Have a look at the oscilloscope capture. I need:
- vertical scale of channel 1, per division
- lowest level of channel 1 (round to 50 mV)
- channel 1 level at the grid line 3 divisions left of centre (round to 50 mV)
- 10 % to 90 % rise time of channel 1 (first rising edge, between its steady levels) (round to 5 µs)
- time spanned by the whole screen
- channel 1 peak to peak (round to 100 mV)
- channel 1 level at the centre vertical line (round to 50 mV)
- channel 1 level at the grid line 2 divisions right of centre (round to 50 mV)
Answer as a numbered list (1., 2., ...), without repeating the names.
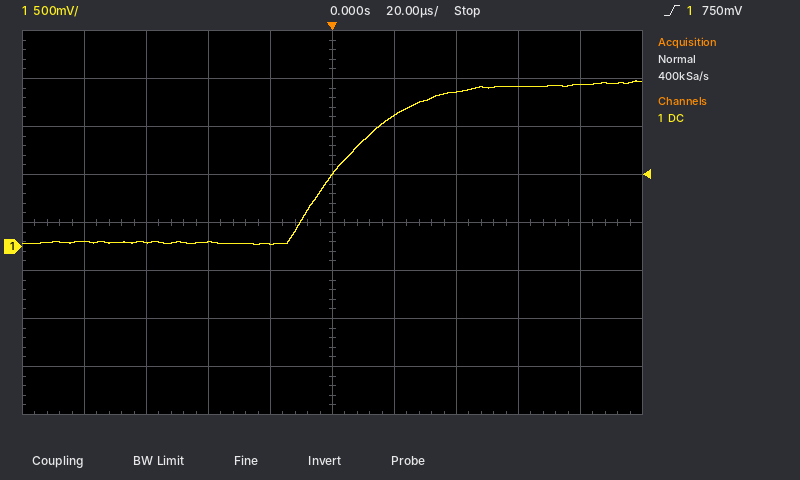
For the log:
1. 500 mV
2. 0 mV
3. 50 mV
4. 40 µs
5. 200 µs
6. 1.70 V
7. 750 mV
8. 1.60 V
